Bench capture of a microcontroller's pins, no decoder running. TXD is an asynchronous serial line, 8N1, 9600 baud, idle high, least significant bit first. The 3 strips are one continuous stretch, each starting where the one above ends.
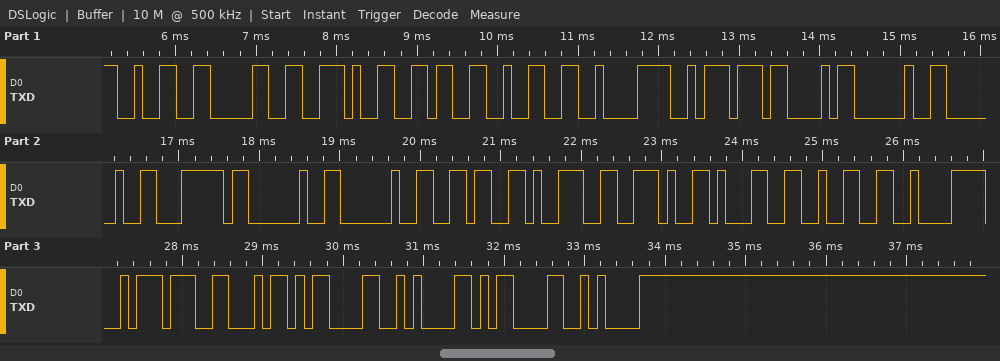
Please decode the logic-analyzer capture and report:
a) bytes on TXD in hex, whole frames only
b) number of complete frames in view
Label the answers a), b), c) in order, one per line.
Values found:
a) 32 30 2E 36 32 C2 BA 43 20 20 7C 20 20 36 39 2E 31 32 C2 BA 46 0D 0A 0D 0A
b) 25
